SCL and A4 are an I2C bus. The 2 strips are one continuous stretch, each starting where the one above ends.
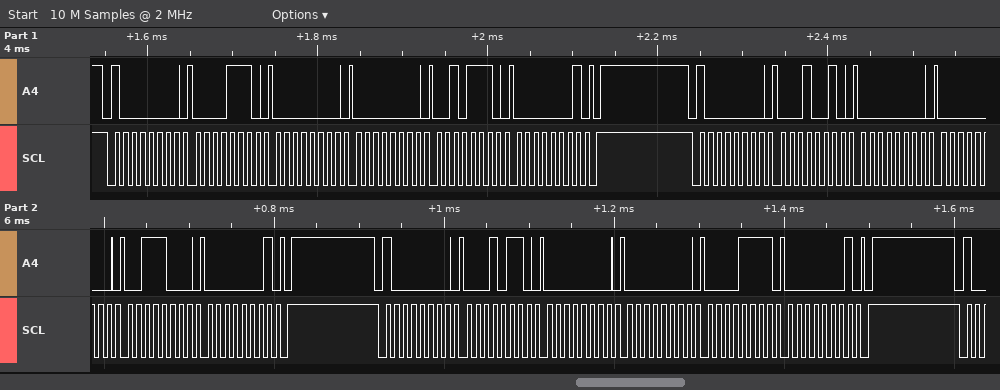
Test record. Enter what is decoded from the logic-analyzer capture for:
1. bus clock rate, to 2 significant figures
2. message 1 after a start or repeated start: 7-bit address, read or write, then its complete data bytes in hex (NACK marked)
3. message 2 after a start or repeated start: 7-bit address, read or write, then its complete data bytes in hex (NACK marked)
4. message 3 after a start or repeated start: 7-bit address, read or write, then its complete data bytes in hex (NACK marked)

100 kHz
0x40 write: 0E 00 00 2E 01
0x40 write: 12 00 00 38 01
0x40 write: 16 00 00 0F 01
